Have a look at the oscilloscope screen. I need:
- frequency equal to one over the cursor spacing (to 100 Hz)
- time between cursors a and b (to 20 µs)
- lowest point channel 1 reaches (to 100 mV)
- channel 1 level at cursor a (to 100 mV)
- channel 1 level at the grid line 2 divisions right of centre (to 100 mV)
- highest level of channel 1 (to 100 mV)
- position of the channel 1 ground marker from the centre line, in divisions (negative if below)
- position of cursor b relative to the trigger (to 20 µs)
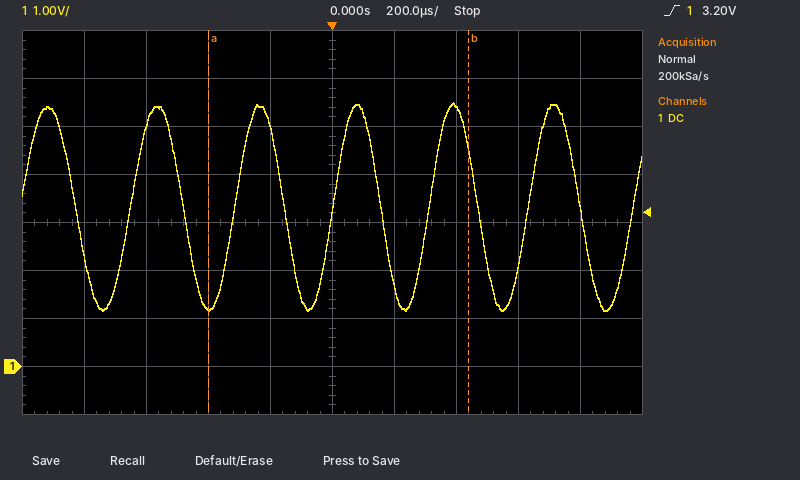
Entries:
1.2 kHz
840 µs
1.2 V
1.2 V
5.4 V
5.5 V
-3.0 div
+440 µs
